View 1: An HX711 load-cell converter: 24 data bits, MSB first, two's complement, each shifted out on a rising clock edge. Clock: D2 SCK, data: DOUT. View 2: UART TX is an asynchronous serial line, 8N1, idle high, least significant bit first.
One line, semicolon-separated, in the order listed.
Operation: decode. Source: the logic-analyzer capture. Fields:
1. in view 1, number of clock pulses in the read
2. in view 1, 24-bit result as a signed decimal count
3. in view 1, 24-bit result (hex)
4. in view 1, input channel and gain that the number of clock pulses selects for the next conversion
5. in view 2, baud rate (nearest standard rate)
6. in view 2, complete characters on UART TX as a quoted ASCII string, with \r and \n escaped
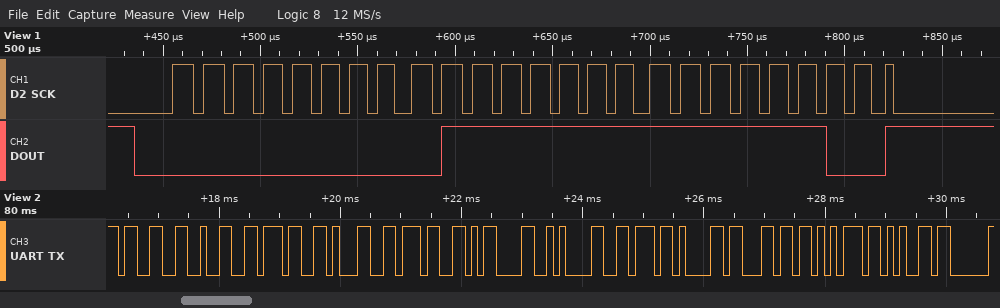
25; 32764; 0x007FFC; channel A, gain 128; 9600 baud; "32717\r\nvalue"
